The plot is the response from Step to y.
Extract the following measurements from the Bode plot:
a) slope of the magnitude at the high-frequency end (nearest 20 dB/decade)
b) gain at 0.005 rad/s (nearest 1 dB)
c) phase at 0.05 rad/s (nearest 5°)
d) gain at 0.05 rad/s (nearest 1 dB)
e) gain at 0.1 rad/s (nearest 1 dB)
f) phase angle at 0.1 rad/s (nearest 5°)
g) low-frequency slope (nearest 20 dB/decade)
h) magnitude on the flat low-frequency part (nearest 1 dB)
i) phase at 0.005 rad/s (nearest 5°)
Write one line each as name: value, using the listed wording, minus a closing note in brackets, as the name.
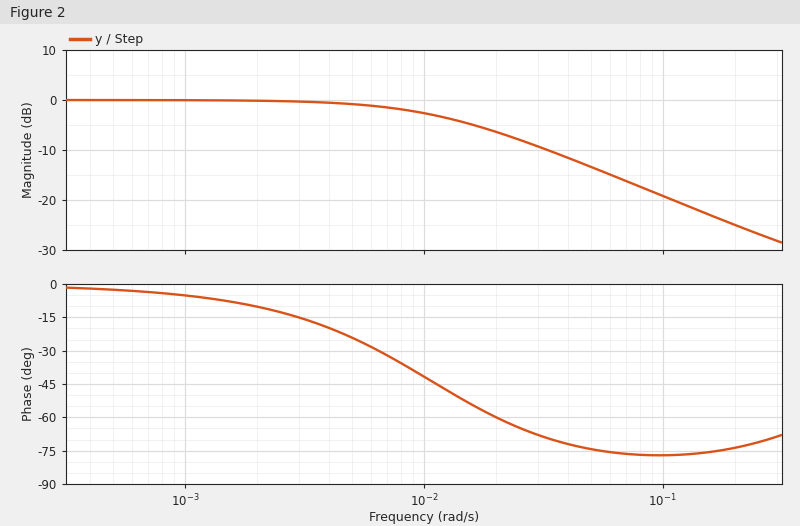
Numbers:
slope of the magnitude at the high-frequency end: -20 dB/decade
gain at 0.005 rad/s: -1 dB
phase at 0.05 rad/s: -75°
gain at 0.05 rad/s: -13 dB
gain at 0.1 rad/s: -19 dB
phase angle at 0.1 rad/s: -75°
low-frequency slope: 0 dB/decade
magnitude on the flat low-frequency part: 0 dB
phase at 0.005 rad/s: -25°
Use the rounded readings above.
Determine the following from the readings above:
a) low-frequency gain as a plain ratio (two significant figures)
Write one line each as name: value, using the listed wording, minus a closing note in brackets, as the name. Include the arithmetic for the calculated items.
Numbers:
low-frequency gain as a plain ratio: 10^(0 / 20) = 1.0
